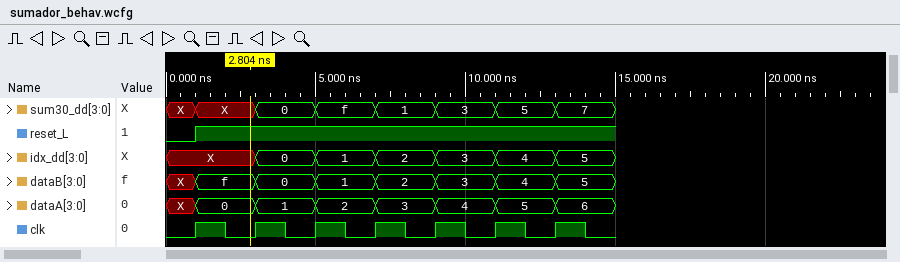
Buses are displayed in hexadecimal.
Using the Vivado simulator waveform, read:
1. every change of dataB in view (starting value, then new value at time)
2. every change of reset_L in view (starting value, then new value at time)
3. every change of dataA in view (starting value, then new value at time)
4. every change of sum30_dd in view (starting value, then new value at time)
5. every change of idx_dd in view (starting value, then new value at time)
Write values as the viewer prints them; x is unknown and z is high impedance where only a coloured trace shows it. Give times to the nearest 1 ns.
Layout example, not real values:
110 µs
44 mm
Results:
X, f at 1 ns, 0 at 3 ns, 1 at 5 ns, 2 at 7 ns, 3 at 9 ns, 4 at 11 ns, 5 at 13 ns
0, 1 at 1 ns
X, 0 at 1 ns, 1 at 3 ns, 2 at 5 ns, 3 at 7 ns, 4 at 9 ns, 5 at 11 ns, 6 at 13 ns
X, X at 1 ns, 0 at 3 ns, f at 5 ns, 1 at 7 ns, 3 at 9 ns, 5 at 11 ns, 7 at 13 ns
X, 0 at 3 ns, 1 at 5 ns, 2 at 7 ns, 3 at 9 ns, 4 at 11 ns, 5 at 13 ns
